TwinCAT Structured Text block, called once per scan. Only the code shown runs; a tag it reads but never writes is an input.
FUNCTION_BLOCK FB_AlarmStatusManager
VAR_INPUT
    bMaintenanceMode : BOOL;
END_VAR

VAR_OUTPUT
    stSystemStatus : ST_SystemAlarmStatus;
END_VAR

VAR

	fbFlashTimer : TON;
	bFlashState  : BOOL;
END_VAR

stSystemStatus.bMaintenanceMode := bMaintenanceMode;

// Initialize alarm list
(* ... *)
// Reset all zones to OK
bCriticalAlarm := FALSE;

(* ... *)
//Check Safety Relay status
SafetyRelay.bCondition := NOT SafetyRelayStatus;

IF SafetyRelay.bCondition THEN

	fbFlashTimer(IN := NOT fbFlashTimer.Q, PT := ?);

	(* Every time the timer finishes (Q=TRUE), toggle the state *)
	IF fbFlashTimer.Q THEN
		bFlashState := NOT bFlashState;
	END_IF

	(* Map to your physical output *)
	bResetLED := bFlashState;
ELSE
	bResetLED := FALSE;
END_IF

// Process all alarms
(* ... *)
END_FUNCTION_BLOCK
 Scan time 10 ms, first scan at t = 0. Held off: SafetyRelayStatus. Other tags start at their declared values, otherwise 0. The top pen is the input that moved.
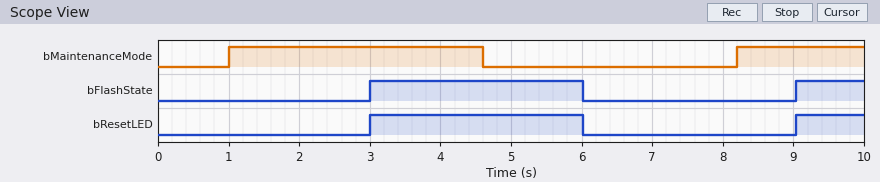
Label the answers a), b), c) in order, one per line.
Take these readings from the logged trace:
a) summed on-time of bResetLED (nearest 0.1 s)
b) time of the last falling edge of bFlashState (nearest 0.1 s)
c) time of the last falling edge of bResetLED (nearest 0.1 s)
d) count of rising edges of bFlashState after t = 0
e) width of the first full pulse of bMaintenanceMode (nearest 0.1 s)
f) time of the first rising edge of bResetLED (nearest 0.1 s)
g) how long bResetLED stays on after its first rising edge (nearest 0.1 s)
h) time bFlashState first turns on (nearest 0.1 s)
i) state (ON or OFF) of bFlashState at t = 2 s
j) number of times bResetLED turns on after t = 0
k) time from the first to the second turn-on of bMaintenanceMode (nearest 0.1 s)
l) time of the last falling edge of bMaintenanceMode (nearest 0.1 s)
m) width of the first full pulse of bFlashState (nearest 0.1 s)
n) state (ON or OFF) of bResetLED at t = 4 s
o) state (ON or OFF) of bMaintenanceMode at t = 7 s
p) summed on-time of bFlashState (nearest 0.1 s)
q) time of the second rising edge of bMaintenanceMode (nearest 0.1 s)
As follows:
a) 4.0 s
b) 6.0 s
c) 6.0 s
d) 2
e) 3.6 s
f) 3.0 s
g) 3.0 s
h) 3.0 s
i) OFF
j) 2
k) 7.2 s
l) 4.6 s
m) 3.0 s
n) ON
o) OFF
p) 4.0 s
q) 8.2 s
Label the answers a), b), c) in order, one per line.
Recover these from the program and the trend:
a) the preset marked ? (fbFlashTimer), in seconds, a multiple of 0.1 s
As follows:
a) 3.0 s
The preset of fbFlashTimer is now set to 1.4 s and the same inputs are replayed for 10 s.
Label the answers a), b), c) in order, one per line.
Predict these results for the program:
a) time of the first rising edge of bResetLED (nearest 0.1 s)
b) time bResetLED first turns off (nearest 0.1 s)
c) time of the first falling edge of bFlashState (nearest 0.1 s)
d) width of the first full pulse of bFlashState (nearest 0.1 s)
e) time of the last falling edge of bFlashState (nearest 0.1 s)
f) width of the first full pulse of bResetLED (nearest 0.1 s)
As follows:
a) 1.4 s
b) 2.8 s
c) 2.8 s
d) 1.4 s
e) 8.5 s
f) 1.4 s
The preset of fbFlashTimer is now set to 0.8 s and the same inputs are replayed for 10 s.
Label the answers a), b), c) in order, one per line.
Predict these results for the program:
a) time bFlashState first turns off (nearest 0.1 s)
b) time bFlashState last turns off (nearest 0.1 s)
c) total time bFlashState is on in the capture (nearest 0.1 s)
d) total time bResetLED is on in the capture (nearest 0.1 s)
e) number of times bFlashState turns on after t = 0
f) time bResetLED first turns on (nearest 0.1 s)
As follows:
a) 1.6 s
b) 9.8 s
c) 4.9 s
d) 4.9 s
e) 6
f) 0.8 s
